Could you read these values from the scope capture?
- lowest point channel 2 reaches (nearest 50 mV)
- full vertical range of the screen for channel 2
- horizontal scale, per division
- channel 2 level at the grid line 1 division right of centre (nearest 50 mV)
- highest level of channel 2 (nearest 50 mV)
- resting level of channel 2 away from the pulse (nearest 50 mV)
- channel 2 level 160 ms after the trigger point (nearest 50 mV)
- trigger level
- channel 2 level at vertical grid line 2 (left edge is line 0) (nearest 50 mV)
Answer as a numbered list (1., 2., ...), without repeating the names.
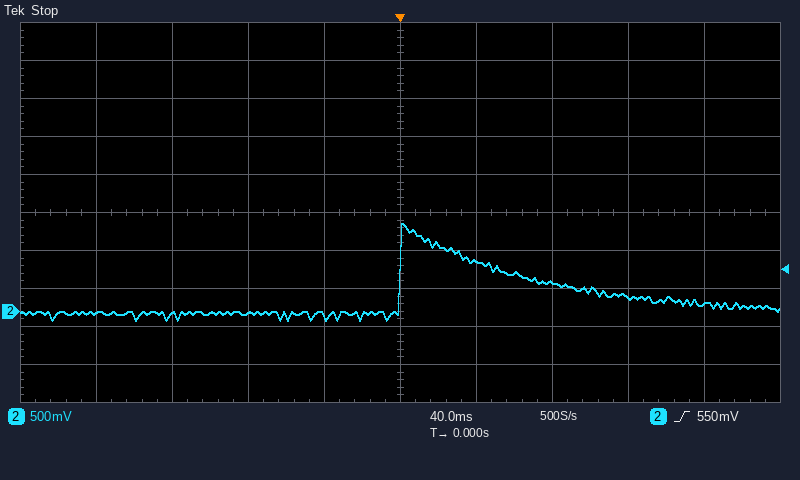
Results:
1. -100 mV
2. 5 V
3. 40 ms
4. 650 mV
5. 1.15 V
6. 0 mV
7. 100 mV
8. 550 mV
9. -50 mV
